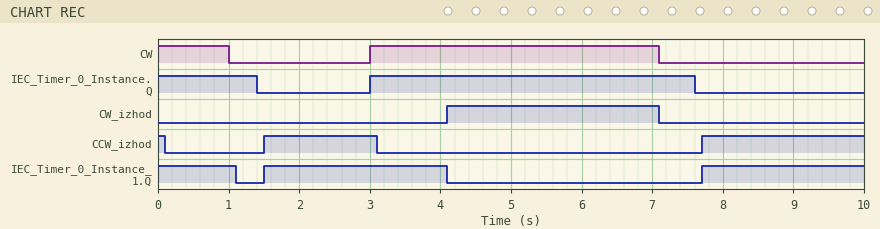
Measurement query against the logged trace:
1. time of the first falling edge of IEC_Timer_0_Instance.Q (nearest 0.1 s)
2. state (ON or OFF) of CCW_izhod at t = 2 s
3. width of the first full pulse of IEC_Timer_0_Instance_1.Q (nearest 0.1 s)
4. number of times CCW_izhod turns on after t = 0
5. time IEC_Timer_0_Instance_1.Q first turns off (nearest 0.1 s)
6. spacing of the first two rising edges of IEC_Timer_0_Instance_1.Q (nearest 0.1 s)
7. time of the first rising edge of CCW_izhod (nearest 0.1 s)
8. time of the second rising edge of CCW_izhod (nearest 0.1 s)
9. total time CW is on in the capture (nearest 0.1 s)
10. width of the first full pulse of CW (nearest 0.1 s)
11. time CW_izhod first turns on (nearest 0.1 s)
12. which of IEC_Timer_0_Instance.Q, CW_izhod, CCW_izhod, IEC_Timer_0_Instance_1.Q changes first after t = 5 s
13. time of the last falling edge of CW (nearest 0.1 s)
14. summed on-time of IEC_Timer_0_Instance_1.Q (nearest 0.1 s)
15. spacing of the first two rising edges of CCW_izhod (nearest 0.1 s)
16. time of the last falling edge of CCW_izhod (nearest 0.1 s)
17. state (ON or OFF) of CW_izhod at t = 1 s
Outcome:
1.4 s
ON
2.6 s
2
1.1 s
6.2 s
1.5 s
7.7 s
5.1 s
4.1 s
4.1 s
CW_izhod
7.1 s
6.0 s
6.2 s
3.1 s
OFF
